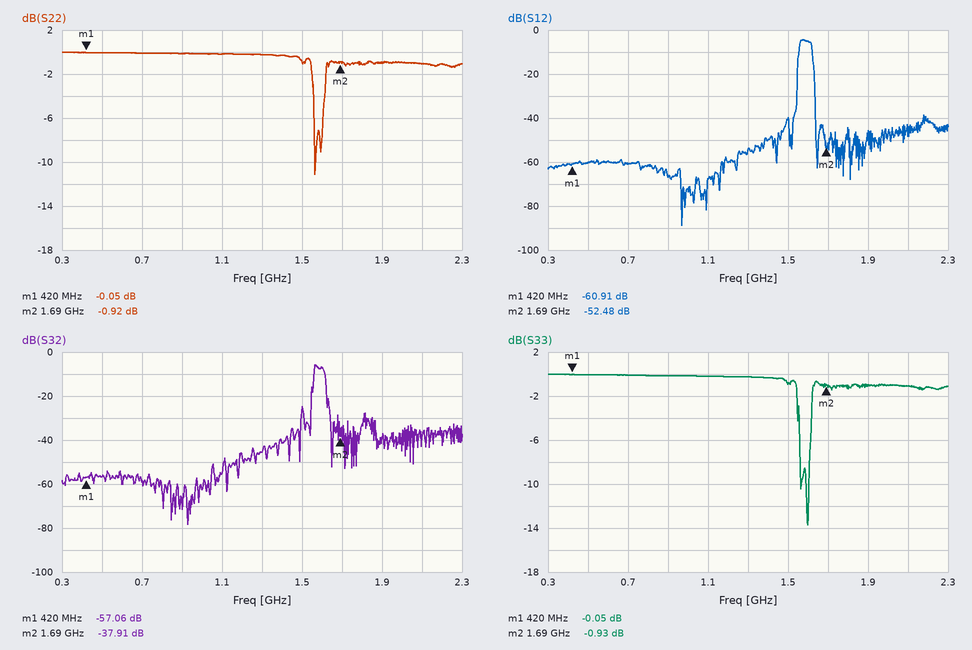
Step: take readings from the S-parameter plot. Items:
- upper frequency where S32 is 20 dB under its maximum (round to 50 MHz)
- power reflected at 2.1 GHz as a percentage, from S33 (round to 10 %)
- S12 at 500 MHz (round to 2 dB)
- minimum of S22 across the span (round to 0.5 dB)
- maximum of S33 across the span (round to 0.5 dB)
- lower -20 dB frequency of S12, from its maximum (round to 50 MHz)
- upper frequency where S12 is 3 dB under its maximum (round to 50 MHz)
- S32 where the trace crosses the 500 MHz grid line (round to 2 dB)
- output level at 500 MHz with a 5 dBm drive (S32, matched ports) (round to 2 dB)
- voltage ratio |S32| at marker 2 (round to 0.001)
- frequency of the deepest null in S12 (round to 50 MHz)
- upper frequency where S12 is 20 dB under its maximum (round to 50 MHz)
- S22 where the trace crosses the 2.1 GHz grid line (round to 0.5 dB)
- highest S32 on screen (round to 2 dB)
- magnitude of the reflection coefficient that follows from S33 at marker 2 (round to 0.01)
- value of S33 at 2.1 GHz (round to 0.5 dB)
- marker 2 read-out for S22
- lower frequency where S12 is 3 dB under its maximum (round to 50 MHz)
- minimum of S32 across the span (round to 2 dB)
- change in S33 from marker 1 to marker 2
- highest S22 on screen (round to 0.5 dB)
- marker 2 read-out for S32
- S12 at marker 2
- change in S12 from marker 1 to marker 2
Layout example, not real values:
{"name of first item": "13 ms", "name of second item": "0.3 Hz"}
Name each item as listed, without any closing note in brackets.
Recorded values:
{"upper frequency where S32 is 20 dB under its maximum": "1.65 GHz", "power reflected at 2.1 GHz as a percentage, from S33": "80 %", "S12 at 500 MHz": "-60 dB", "minimum of S22 across the span": "-11.0 dB", "maximum of S33 across the span": "0.0 dB", "lower -20 dB frequency of S12, from its maximum": "1.55 GHz", "upper frequency where S12 is 3 dB under its maximum": "1.60 GHz", "S32 where the trace crosses the 500 MHz grid line": "-56 dB", "output level at 500 MHz with a 5 dBm drive (S32, matched ports)": "-52 dBm", "voltage ratio |S32| at marker 2": "0.013", "frequency of the deepest null in S12": "950 MHz", "upper frequency where S12 is 20 dB under its maximum": "1.65 GHz", "S22 where the trace crosses the 2.1 GHz grid line": "-1.0 dB", "highest S32 on screen": "-6 dB", "magnitude of the reflection coefficient that follows from S33 at marker 2": "0.90", "value of S33 at 2.1 GHz": "-1.0 dB", "marker 2 read-out for S22": "-0.92 dB", "lower frequency where S12 is 3 dB under its maximum": "1.55 GHz", "minimum of S32 across the span": "-78 dB", "change in S33 from marker 1 to marker 2": "-0.88 dB", "highest S22 on screen": "0.0 dB", "marker 2 read-out for S32": "-37.91 dB", "S12 at marker 2": "-52.48 dB", "change in S12 from marker 1 to marker 2": "8.43 dB"}
